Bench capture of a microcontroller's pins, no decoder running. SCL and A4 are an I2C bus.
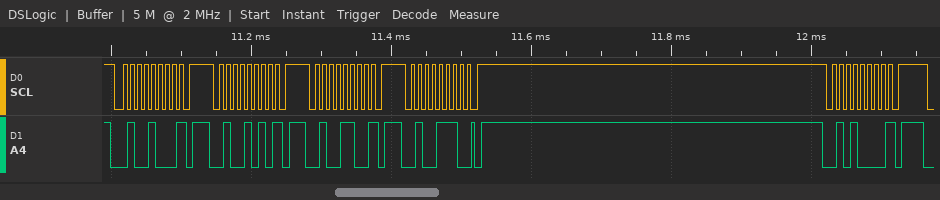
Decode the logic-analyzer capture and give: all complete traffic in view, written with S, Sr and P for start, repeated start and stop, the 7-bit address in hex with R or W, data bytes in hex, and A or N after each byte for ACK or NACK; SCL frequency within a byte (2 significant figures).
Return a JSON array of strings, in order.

["S 24W N P S 25W N P S 26W N P S 27W A P S 28W N P", "100 kHz"]
